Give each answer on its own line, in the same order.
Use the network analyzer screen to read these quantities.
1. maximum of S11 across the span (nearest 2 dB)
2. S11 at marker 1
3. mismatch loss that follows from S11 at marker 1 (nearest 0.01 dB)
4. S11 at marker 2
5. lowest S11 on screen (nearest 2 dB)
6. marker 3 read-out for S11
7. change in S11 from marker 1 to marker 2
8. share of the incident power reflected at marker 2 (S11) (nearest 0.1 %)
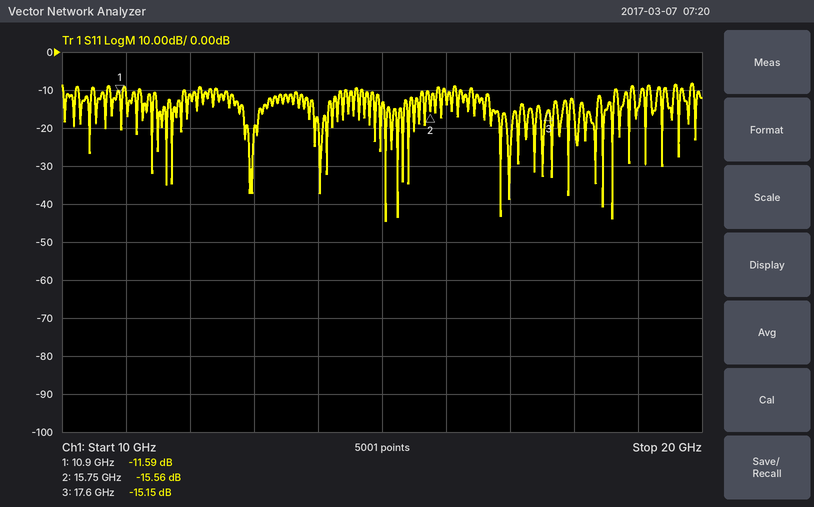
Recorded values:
-8 dB
-11.59 dB
0.31 dB
-15.56 dB
-44 dB
-15.15 dB
-3.97 dB
2.8 %
